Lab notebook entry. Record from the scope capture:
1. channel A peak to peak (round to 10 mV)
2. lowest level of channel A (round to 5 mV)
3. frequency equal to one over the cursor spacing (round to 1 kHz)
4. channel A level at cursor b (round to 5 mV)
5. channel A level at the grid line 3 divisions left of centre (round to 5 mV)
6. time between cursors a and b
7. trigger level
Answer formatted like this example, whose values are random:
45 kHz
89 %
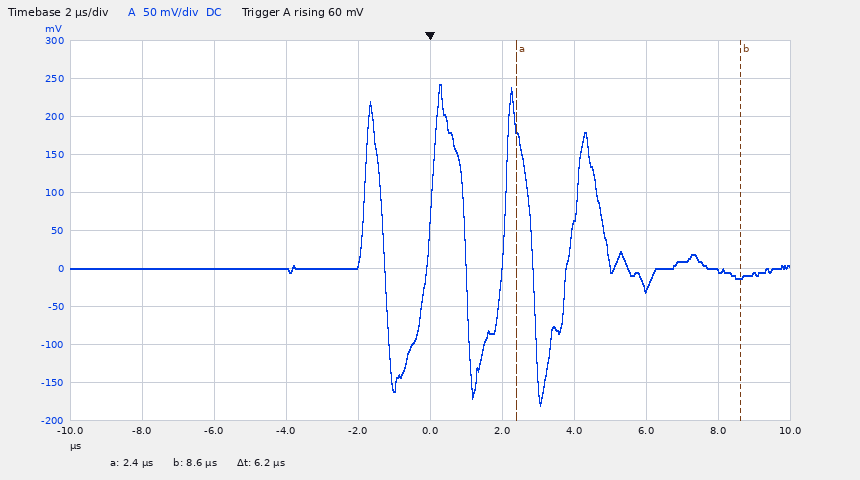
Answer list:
420 mV
-180 mV
161 kHz
-10 mV
0 mV
6.2 µs
60 mV
